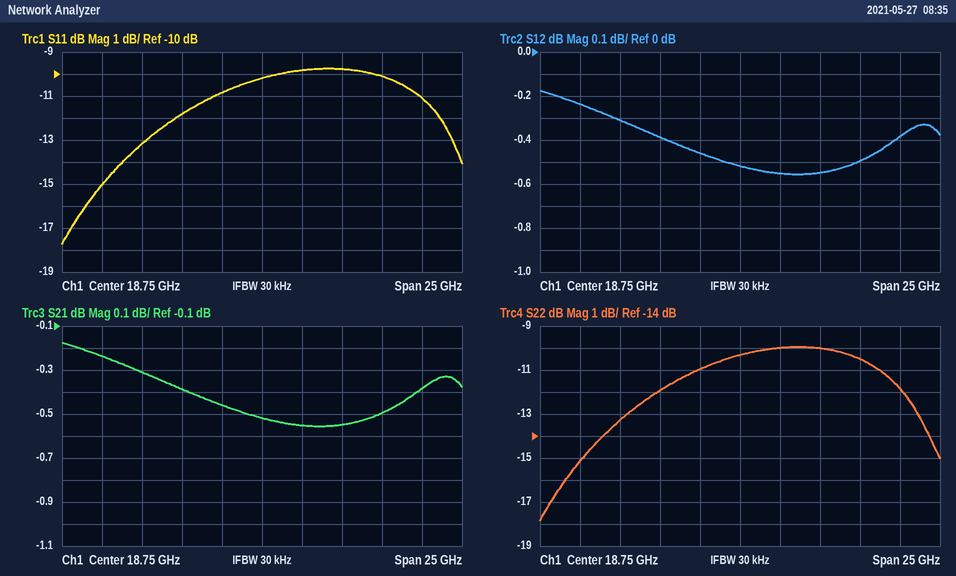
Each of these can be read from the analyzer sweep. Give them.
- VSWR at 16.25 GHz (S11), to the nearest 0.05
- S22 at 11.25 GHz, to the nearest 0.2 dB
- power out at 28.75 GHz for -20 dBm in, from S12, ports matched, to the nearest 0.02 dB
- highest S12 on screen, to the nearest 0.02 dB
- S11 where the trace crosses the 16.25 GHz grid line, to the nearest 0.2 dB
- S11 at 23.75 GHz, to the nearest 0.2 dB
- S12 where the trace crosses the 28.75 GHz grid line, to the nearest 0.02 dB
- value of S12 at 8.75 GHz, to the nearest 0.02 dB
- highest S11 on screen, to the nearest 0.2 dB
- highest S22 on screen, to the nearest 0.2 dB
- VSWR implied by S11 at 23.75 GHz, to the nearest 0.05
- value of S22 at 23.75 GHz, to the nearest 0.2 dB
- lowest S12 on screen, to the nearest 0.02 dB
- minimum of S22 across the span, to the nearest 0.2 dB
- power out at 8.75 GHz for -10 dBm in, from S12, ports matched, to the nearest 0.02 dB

1.80
-13.2 dB
-20.38 dBm
-0.18 dB
-10.8 dB
-9.8 dB
-0.38 dB
-0.24 dB
-9.8 dB
-10.0 dB
1.95
-10.0 dB
-0.56 dB
-17.8 dB
-10.24 dBm
